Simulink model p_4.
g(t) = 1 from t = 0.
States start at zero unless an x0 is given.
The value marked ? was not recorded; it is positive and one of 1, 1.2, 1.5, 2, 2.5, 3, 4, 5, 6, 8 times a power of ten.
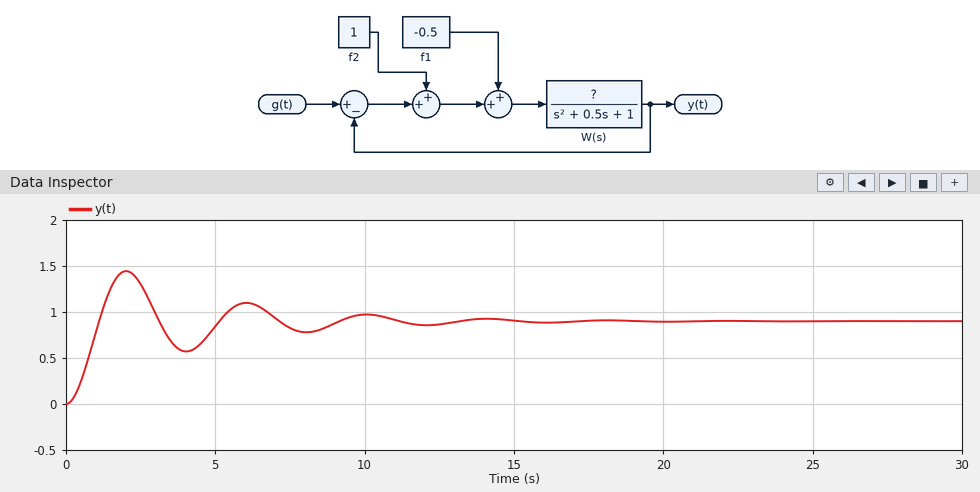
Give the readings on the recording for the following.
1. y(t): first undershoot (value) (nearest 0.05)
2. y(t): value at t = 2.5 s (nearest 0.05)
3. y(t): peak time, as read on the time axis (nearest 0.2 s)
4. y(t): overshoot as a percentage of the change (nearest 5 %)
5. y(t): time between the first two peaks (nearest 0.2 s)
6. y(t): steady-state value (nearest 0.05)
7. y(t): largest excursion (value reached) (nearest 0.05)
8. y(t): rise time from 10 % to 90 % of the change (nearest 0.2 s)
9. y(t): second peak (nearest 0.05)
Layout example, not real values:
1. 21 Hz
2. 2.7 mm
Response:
1. 0.55
2. 1.30
3. 2.0 s
4. 60 %
5. 4.0 s
6. 0.90
7. 1.45
8. 0.8 s
9. 1.10
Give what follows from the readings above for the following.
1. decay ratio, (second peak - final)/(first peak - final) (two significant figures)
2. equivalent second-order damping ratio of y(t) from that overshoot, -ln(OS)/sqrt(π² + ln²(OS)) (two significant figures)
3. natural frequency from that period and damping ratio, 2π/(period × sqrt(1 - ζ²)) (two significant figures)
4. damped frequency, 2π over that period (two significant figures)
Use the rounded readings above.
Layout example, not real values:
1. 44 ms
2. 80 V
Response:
1. 0.36
2. 0.16
3. 1.6 rad/s
4. 1.6 rad/s
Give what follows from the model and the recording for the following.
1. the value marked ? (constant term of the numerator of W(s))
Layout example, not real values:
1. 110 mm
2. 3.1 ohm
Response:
1. 1.5
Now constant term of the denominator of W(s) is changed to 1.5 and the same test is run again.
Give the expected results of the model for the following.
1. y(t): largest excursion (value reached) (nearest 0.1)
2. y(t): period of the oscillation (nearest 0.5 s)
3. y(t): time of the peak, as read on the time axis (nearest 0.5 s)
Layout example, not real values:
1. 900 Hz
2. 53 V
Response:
1. 1.2
2. 3.5 s
3. 2.0 s
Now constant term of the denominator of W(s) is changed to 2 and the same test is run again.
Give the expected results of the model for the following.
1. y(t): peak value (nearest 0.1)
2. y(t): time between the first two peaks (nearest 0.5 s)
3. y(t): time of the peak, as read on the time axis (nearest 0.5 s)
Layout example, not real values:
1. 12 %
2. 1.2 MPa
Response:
1. 1.1
2. 3.5 s
3. 1.5 s
